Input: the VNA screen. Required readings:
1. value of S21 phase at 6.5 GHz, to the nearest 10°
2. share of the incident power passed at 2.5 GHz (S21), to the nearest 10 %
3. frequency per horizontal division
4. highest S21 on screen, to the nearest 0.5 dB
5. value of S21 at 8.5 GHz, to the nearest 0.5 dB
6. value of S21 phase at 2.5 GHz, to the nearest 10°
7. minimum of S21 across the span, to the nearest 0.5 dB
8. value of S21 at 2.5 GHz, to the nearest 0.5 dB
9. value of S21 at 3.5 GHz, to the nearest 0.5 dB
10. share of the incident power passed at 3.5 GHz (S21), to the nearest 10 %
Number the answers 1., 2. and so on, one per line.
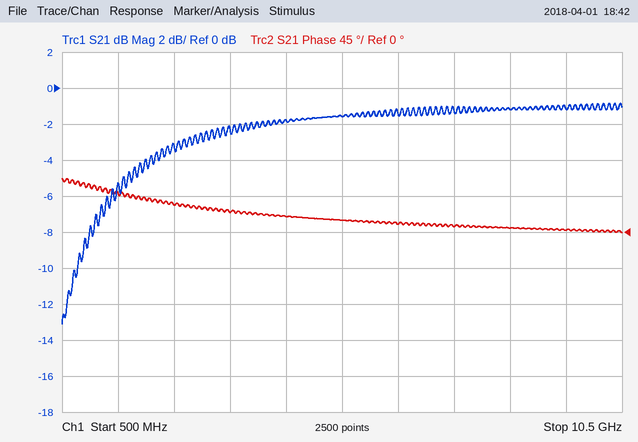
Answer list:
1. 10°
2. 50 %
3. 1 GHz
4. -1.0 dB
5. -1.0 dB
6. 30°
7. -13.0 dB
8. -3.0 dB
9. -2.5 dB
10. 60 %
